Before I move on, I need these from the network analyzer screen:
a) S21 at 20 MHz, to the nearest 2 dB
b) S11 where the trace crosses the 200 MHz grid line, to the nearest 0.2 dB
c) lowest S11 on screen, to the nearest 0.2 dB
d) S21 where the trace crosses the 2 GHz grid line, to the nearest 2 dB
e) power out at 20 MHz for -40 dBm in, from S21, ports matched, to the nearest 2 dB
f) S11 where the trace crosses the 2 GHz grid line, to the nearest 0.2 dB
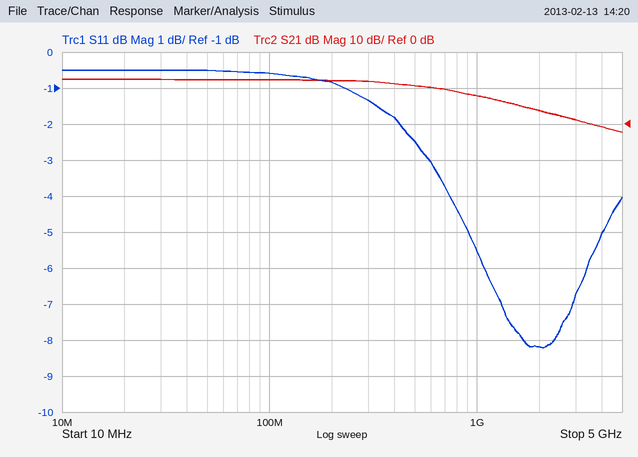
12 dB
-0.8 dB
-8.2 dB
4 dB
-28 dBm
-8.2 dB
